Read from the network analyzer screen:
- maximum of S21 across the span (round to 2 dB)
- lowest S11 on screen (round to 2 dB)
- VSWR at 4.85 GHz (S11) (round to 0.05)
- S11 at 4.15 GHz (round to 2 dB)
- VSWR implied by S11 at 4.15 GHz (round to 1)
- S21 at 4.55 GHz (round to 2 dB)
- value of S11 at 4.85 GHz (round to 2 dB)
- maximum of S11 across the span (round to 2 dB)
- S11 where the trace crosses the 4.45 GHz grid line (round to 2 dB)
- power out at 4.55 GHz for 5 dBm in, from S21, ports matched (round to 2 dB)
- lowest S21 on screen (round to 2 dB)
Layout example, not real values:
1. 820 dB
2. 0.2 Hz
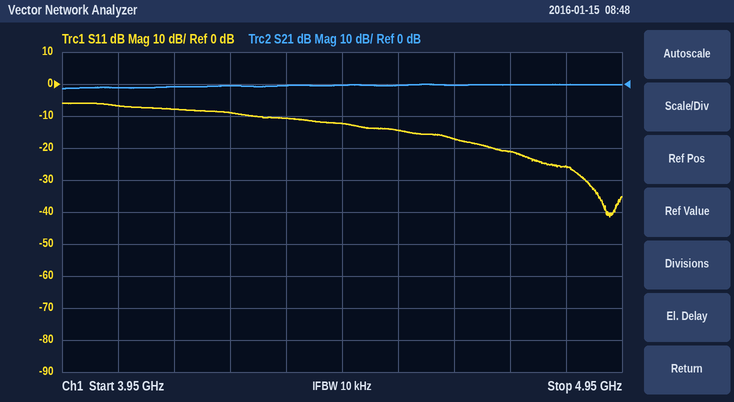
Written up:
1. 0 dB
2. -42 dB
3. 1.10
4. -8 dB
5. 2
6. 0 dB
7. -26 dB
8. -6 dB
9. -12 dB
10. 4 dBm
11. -2 dB
